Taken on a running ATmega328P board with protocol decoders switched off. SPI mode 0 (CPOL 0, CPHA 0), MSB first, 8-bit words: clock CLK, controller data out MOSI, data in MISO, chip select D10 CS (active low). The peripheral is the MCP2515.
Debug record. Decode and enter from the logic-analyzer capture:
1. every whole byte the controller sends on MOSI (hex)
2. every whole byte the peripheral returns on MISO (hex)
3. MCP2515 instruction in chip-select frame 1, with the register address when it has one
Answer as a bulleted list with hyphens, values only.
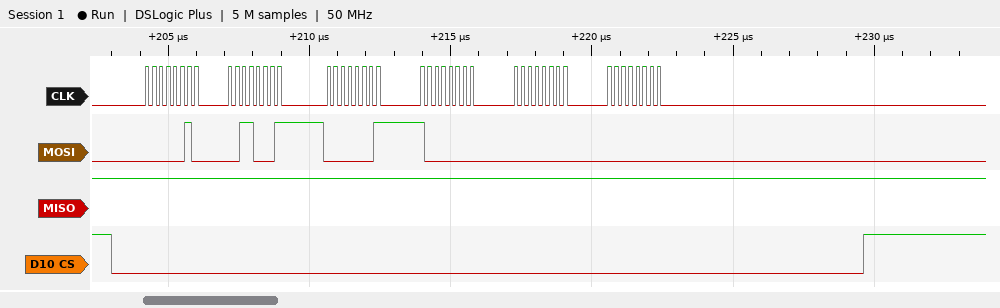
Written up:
- 02 31 01 80 00 00
- FF FF FF FF FF FF
- WRITE 0x31
